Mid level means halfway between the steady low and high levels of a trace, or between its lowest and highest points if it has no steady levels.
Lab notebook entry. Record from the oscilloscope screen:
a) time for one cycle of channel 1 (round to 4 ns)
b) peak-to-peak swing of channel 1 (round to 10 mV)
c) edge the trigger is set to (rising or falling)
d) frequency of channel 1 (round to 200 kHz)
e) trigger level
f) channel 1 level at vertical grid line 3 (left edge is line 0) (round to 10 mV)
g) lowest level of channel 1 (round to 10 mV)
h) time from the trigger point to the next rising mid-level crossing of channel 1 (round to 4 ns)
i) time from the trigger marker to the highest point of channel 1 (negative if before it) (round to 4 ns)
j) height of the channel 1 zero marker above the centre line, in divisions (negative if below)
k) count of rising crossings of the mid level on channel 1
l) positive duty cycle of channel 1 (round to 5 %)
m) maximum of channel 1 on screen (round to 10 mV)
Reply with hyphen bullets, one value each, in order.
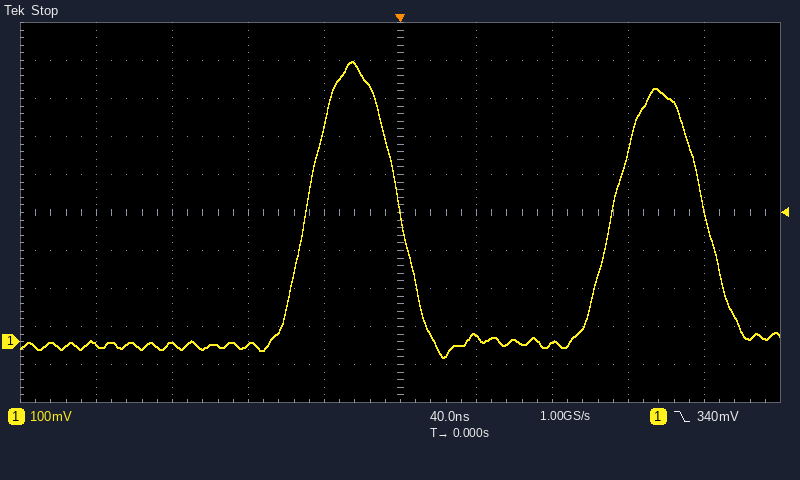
- 160 ns
- 780 mV
- falling
- 6.2 MHz
- 340 mV
- -10 mV
- -40 mV
- 112 ns
- -24 ns
- -3.4 div
- 2
- 30 %
- 740 mV
